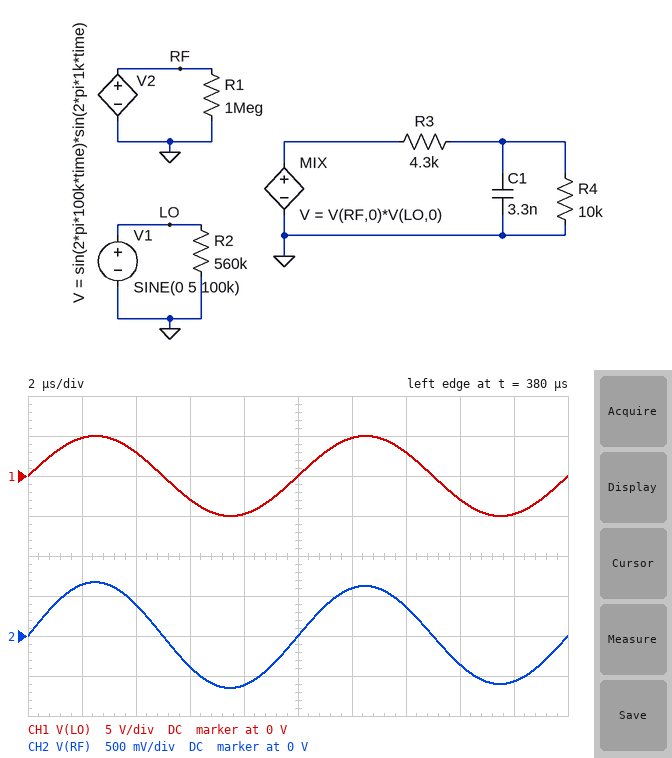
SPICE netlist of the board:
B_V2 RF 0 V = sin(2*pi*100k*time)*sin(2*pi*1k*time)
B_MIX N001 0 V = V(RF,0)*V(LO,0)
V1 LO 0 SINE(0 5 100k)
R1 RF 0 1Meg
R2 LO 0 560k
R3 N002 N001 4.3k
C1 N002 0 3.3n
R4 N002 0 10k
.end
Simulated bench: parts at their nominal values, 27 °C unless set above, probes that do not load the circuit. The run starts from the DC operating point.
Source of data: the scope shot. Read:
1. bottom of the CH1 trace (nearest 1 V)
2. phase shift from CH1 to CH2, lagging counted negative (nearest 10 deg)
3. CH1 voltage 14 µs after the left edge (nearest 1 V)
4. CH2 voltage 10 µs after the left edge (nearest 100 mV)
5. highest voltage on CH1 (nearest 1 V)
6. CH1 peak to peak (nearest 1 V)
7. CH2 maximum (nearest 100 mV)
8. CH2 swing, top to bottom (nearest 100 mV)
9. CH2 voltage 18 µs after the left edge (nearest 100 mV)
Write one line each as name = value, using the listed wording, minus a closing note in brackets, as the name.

bottom of the CH1 trace = -5 V
phase shift from CH1 to CH2, lagging counted negative = 0 deg
CH1 voltage 14 µs after the left edge = 3 V
CH2 voltage 10 µs after the left edge = 0 V
highest voltage on CH1 = 5 V
CH1 peak to peak = 10 V
CH2 maximum = 700 mV
CH2 swing, top to bottom = 1.3 V
CH2 voltage 18 µs after the left edge = -600 mV
